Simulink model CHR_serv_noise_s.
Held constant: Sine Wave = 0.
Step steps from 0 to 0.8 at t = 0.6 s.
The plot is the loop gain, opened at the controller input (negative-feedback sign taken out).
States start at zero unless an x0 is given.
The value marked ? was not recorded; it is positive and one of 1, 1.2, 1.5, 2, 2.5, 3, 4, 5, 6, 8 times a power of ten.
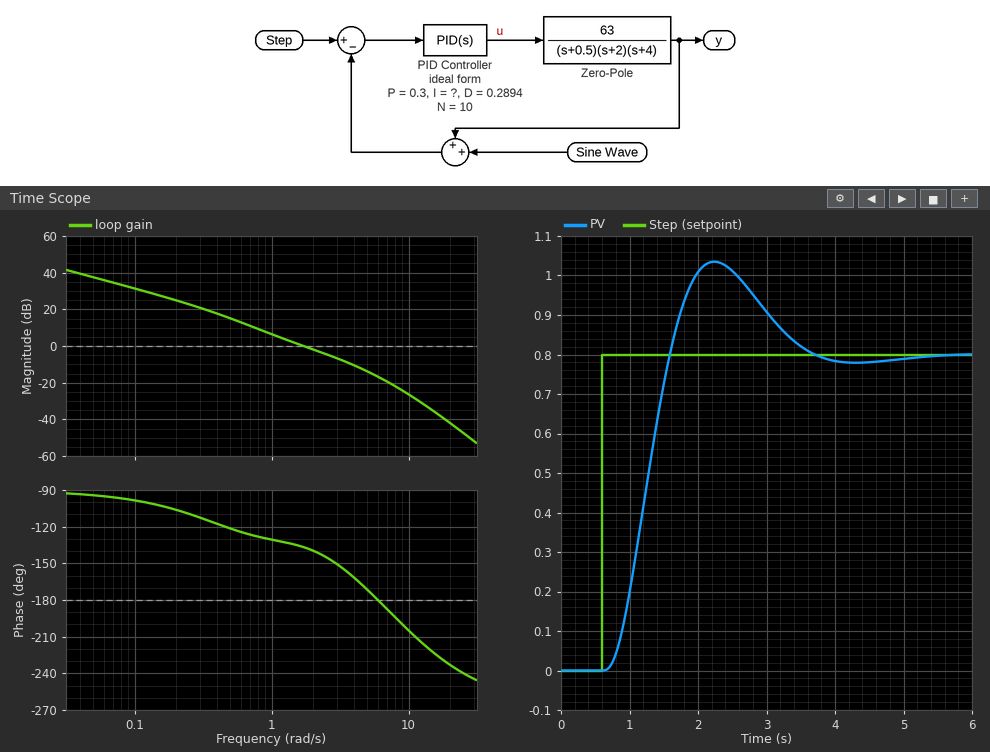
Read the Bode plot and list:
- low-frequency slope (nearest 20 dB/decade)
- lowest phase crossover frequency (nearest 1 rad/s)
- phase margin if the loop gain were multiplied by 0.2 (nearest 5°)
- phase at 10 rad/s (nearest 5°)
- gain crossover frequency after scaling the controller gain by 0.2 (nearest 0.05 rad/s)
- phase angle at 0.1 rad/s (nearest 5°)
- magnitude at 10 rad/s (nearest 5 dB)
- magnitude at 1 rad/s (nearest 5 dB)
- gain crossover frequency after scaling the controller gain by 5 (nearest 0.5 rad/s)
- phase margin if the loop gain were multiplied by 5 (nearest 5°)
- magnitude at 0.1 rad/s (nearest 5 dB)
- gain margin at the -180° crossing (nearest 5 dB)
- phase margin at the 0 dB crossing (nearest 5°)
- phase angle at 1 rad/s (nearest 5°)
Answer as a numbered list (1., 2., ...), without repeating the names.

1. -20 dB/decade
2. 6 rad/s
3. 55°
4. -205°
5. 0.55 rad/s
6. -100°
7. -25 dB
8. 5 dB
9. 5.0 rad/s
10. 10°
11. 30 dB
12. 15 dB
13. 45°
14. -130°
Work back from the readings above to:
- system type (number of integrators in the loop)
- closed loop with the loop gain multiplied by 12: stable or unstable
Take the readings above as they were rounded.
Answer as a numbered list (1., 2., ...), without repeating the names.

1. 1
2. unstable
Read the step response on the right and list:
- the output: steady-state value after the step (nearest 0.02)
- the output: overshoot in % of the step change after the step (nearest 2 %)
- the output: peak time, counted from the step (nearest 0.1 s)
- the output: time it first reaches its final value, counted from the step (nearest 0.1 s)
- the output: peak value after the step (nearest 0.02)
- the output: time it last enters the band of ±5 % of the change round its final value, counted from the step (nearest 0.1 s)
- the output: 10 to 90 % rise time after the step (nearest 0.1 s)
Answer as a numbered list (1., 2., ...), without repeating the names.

1. 0.80
2. 30 %
3. 1.6 s
4. 1.0 s
5. 1.04
6. 2.8 s
7. 0.6 s
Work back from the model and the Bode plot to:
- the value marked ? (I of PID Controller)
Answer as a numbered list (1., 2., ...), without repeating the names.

1. 0.8
